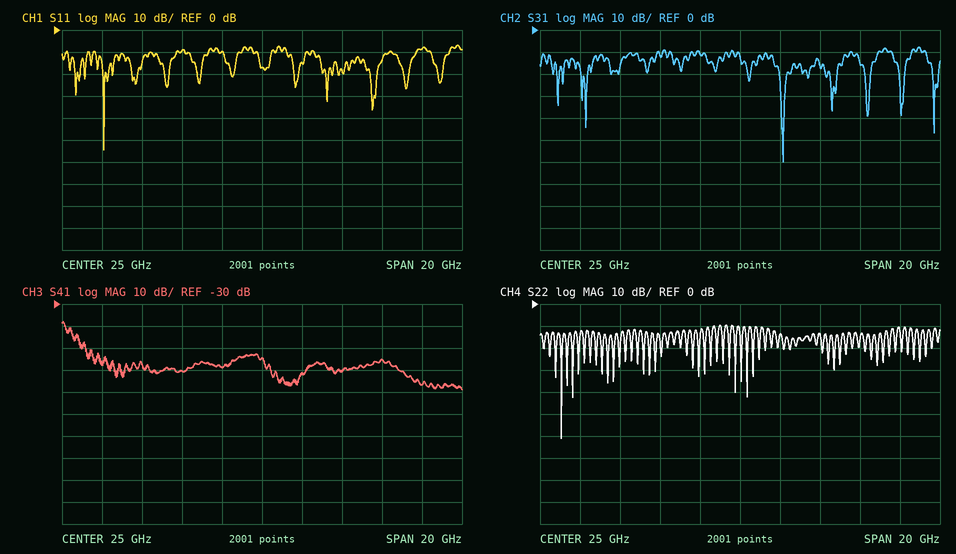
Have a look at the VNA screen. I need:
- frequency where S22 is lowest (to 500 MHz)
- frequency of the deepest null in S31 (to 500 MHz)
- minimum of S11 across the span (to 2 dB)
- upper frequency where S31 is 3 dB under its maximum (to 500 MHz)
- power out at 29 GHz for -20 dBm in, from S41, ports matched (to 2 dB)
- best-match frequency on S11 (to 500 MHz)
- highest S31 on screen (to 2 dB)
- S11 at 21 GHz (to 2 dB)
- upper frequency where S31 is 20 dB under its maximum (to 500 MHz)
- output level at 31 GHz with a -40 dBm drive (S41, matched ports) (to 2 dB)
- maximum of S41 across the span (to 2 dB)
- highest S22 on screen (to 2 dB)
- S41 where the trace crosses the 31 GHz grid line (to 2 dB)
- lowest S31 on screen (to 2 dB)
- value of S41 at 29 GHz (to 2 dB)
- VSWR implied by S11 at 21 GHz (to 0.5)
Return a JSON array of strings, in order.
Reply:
["16.0 GHz", "27.0 GHz", "-54 dB", "34.5 GHz", "-80 dBm", "17.0 GHz", "-8 dB", "-10 dB", "34.5 GHz", "-96 dBm", "-38 dB", "-10 dB", "-56 dB", "-60 dB", "-60 dB", "2.0"]
